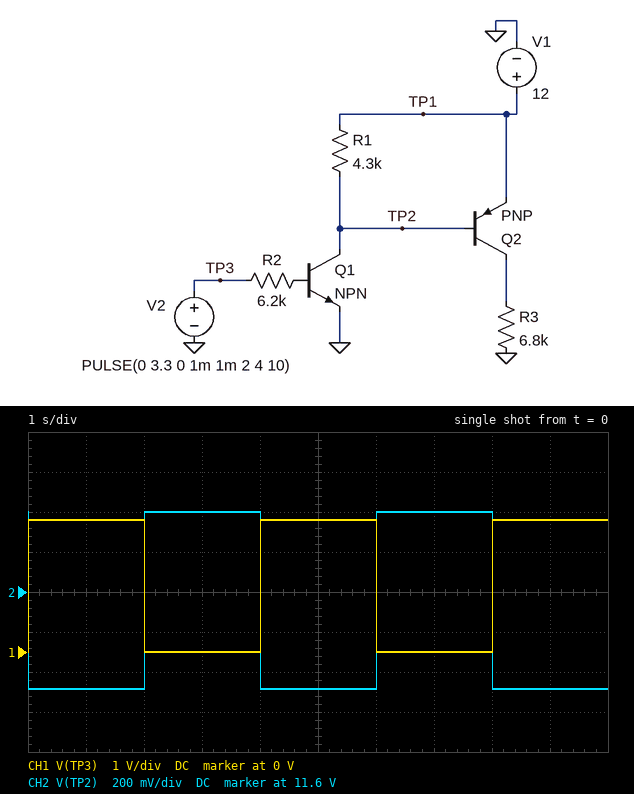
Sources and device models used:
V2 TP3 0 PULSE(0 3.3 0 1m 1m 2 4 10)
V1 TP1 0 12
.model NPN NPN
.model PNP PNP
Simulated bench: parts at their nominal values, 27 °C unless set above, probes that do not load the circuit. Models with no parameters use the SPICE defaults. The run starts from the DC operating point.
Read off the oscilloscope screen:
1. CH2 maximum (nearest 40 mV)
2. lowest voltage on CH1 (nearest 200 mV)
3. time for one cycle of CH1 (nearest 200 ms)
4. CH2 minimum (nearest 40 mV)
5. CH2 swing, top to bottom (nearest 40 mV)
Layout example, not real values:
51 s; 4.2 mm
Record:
12.00 V; 0 V; 4.0 s; 11.12 V; 880 mV
